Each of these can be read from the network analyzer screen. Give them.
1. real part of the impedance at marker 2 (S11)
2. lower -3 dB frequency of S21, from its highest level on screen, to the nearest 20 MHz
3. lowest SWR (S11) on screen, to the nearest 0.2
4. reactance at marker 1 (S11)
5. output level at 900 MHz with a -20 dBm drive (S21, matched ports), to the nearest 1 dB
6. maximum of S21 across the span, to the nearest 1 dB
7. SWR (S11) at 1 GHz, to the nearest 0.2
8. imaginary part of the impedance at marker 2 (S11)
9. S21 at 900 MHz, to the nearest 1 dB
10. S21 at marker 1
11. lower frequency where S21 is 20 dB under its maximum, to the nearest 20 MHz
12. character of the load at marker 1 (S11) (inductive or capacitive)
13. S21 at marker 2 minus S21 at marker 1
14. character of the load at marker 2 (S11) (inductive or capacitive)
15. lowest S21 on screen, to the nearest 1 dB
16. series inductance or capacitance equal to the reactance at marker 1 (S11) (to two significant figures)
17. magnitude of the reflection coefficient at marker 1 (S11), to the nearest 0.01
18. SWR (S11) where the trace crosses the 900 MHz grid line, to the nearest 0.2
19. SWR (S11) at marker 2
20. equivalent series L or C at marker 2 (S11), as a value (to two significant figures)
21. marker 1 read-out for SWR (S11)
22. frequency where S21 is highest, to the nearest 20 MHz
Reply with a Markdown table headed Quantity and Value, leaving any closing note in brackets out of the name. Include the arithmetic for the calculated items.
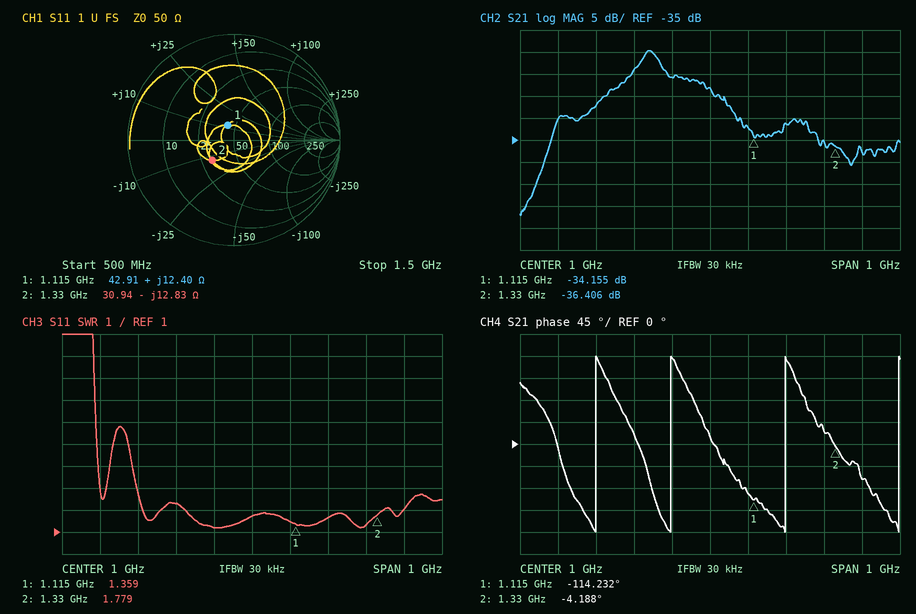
| Quantity | Value |
|---|---|
| real part of the impedance at marker 2 | 30.94 Ω |
| lower -3 dB frequency of S21, from its highest level on screen, to the nearest 20 MHz | 820 MHz |
| lowest SWR (S11) on screen, to the nearest 0.2 | 1.2 |
| reactance at marker 1 | +12.40 Ω |
| output level at 900 MHz with a -20 dBm drive (S21, matched ports), to the nearest 1 dB | -20 dBm + (-21 dB) = -41 dBm |
| maximum of S21 across the span, to the nearest 1 dB | -15 dB |
| SWR (S11) at 1 GHz, to the nearest 0.2 | 1.8 |
| imaginary part of the impedance at marker 2 | -12.83 Ω |
| S21 at 900 MHz, to the nearest 1 dB | -21 dB |
| S21 at marker 1 | -34.155 dB |
| lower frequency where S21 is 20 dB under its maximum, to the nearest 20 MHz | 580 MHz |
| character of the load at marker 1 (S11) | inductive |
| S21 at marker 2 minus S21 at marker 1 | -36.406 − (-34.155) = -2.251 dB |
| character of the load at marker 2 (S11) | capacitive |
| lowest S21 on screen, to the nearest 1 dB | -52 dB |
| series inductance or capacitance equal to the reactance at marker 1 (S11) | L = 12.4 Ω/(2π × 1.115 GHz) ≈ 1.8 nH |
| magnitude of the reflection coefficient at marker 1 (S11), to the nearest 0.01 | 0.15 |
| SWR (S11) where the trace crosses the 900 MHz grid line, to the nearest 0.2 | 1.2 |
| SWR (S11) at marker 2 | 1.779 |
| equivalent series L or C at marker 2 (S11), as a value | C = 1/(2π × 1.33 GHz × 12.83 Ω) ≈ 9.3 pF |
| marker 1 read-out for SWR | 1.359 |
| frequency where S21 is highest, to the nearest 20 MHz | 840 MHz |
